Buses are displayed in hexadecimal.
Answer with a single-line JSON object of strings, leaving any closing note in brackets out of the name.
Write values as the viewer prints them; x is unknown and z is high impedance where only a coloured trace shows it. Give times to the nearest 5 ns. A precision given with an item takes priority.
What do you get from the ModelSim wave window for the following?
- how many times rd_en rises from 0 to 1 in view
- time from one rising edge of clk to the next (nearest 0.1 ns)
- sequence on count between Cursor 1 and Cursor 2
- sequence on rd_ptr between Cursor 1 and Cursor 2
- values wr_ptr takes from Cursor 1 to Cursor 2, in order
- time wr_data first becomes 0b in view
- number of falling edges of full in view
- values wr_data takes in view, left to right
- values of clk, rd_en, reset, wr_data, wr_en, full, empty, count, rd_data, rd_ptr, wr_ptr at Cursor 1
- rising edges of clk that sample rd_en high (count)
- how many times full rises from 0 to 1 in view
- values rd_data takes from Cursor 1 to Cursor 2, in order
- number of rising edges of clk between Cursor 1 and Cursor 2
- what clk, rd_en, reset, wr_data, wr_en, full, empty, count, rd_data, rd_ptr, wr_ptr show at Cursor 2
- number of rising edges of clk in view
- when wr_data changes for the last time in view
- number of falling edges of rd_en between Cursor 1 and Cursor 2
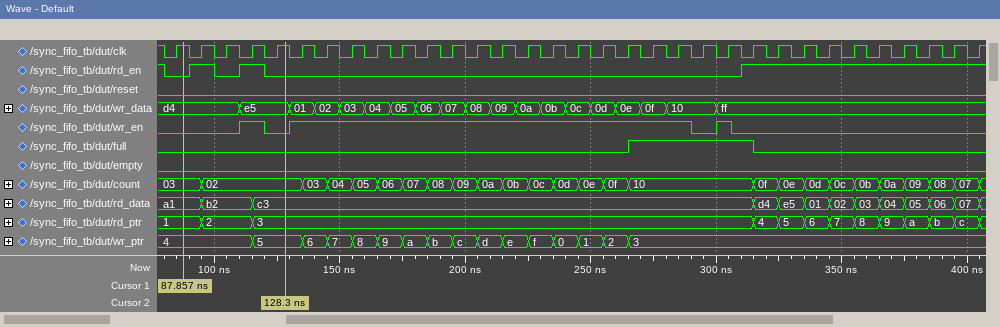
{"how many times rd_en rises from 0 to 1 in view": "3", "time from one rising edge of clk to the next": "10 ns", "sequence on count between Cursor 1 and Cursor 2": "03, 02", "sequence on rd_ptr between Cursor 1 and Cursor 2": "1, 2, 3", "values wr_ptr takes from Cursor 1 to Cursor 2, in order": "4, 5", "time wr_data first becomes 0b in view": "230 ns", "number of falling edges of full in view": "1", "values wr_data takes in view, left to right": "d4, e5, 01, 02, 03, 04, 05, 06, 07, 08, 09, 0a, 0b, 0c, 0d, 0e, 0f, 10, ff", "values of clk, rd_en, reset, wr_data, wr_en, full, empty, count, rd_data, rd_ptr, wr_ptr at Cursor 1": "clk=1, rd_en=0, reset=0, wr_data=d4, wr_en=0, full=0, empty=0, count=03, rd_data=a1, rd_ptr=1, wr_ptr=4", "rising edges of clk that sample rd_en high": "12", "how many times full rises from 0 to 1 in view": "1", "values rd_data takes from Cursor 1 to Cursor 2, in order": "a1, b2, c3", "number of rising edges of clk between Cursor 1 and Cursor 2": "4", "what clk, rd_en, reset, wr_data, wr_en, full, empty, count, rd_data, rd_ptr, wr_ptr show at Cursor 2": "clk=1, rd_en=0, reset=0, wr_data=e5, wr_en=0, full=0, empty=0, count=02, rd_data=c3, rd_ptr=3, wr_ptr=5", "number of rising edges of clk in view": "33", "when wr_data changes for the last time in view": "300 ns", "number of falling edges of rd_en between Cursor 1 and Cursor 2": "2"}
